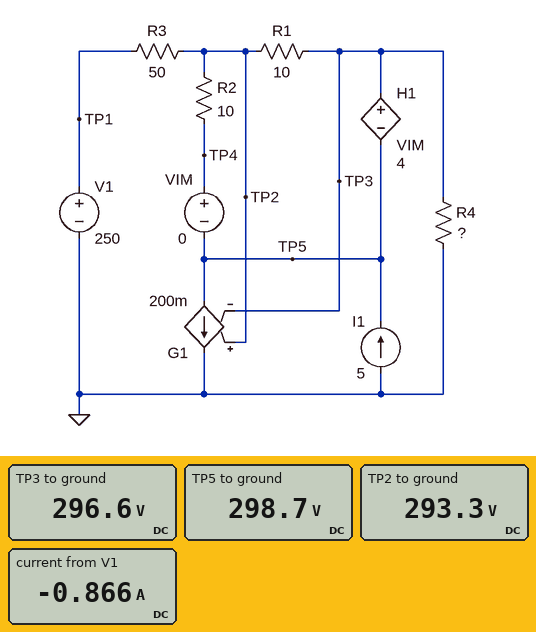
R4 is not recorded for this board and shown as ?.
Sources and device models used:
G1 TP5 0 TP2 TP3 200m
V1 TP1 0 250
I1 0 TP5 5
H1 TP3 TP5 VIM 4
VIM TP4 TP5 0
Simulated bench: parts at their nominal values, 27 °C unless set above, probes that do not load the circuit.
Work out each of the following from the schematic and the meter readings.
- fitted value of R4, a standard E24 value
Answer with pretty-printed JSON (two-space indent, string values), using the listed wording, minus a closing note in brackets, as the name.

{
  "fitted value of R4, a standard E24 value": "62 Ω"
}
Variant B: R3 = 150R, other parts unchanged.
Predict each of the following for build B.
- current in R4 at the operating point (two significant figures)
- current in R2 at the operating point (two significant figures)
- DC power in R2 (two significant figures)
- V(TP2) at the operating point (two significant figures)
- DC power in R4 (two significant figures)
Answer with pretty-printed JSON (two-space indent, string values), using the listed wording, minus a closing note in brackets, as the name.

{
  "current in R4 at the operating point": "4.9 A",
  "current in R2 at the operating point": "220 mA",
  "DC power in R2": "490 mW",
  "V(TP2) at the operating point": "300 V",
  "DC power in R4": "1.5 kW"
}
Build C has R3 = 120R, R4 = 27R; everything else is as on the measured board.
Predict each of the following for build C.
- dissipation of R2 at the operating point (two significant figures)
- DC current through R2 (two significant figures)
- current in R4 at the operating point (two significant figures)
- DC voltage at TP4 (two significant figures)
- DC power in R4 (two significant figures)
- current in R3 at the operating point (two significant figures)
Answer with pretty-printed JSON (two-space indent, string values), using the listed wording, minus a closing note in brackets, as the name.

{
  "dissipation of R2 at the operating point": "3.0 W",
  "DC current through R2": "550 mA",
  "current in R4 at the operating point": "5.2 A",
  "DC voltage at TP4": "140 V",
  "DC power in R4": "740 W",
  "current in R3 at the operating point": "880 mA"
}
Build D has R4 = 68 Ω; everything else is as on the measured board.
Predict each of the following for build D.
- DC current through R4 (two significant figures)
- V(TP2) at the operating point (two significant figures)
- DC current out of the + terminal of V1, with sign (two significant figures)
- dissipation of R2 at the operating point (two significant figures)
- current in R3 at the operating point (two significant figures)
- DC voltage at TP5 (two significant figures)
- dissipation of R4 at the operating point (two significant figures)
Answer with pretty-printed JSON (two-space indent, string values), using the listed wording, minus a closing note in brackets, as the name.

{
  "DC current through R4": "4.7 A",
  "V(TP2) at the operating point": "310 V",
  "DC current out of the + terminal of V1, with sign": "-1.3 A",
  "dissipation of R2 at the operating point": "6.3 W",
  "current in R3 at the operating point": "1.3 A",
  "DC voltage at TP5": "320 V",
  "dissipation of R4 at the operating point": "1.5 kW"
}
